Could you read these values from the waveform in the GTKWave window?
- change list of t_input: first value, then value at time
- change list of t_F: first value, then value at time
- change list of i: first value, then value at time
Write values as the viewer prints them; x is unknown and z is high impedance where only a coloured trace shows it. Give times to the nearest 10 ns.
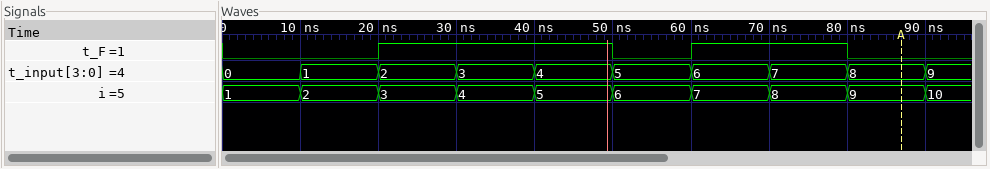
0, 1 at 10 ns, 2 at 20 ns, 3 at 30 ns, 4 at 40 ns, 5 at 50 ns, 6 at 60 ns, 7 at 70 ns, 8 at 80 ns, 9 at 90 ns
0, 1 at 20 ns, 0 at 50 ns, 1 at 60 ns, 0 at 80 ns
1, 2 at 10 ns, 3 at 20 ns, 4 at 30 ns, 5 at 40 ns, 6 at 50 ns, 7 at 60 ns, 8 at 70 ns, 9 at 80 ns, 10 at 90 ns
